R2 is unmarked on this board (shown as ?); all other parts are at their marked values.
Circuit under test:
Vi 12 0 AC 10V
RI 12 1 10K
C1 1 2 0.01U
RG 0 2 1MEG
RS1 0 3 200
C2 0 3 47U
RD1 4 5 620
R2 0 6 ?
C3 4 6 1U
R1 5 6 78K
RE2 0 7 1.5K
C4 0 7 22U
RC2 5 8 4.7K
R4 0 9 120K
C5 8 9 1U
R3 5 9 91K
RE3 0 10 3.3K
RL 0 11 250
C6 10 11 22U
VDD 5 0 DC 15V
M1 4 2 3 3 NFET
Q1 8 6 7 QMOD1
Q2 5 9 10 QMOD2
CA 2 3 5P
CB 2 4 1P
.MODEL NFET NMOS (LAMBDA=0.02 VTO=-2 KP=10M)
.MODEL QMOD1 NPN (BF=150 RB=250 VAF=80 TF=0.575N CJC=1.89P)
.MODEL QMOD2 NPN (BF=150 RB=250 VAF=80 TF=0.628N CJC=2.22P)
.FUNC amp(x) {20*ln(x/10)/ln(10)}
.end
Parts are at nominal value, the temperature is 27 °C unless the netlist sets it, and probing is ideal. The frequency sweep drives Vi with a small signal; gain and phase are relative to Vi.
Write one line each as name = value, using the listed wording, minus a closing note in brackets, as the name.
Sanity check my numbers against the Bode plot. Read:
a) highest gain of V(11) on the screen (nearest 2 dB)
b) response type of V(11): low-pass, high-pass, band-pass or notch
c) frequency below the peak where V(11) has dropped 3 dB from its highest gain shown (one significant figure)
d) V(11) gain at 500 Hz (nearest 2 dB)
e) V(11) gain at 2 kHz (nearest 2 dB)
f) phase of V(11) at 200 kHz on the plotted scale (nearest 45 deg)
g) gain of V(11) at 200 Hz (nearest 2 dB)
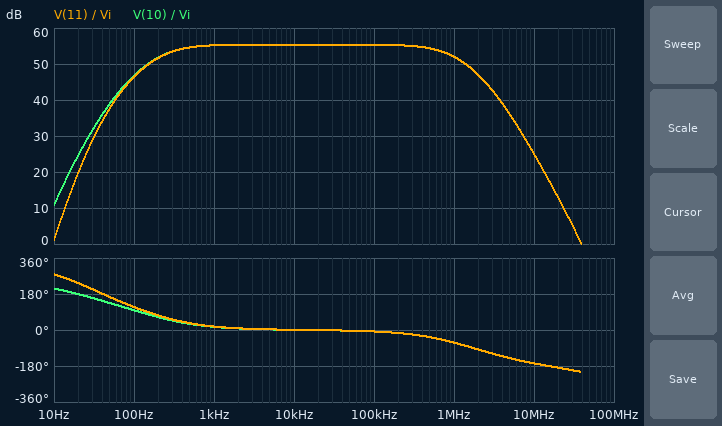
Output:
highest gain of V(11) on the screen = 56 dB
response type of V(11): low-pass, high-pass, band-pass or notch = band-pass
frequency below the peak where V(11) has dropped 3 dB from its highest gain shown = 200 Hz
V(11) gain at 500 Hz = 54 dB
V(11) gain at 2 kHz = 56 dB
phase of V(11) at 200 kHz on the plotted scale = 0 deg
gain of V(11) at 200 Hz = 52 dB
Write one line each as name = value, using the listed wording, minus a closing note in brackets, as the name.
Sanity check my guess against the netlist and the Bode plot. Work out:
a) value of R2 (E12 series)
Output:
value of R2 = 12 kΩ
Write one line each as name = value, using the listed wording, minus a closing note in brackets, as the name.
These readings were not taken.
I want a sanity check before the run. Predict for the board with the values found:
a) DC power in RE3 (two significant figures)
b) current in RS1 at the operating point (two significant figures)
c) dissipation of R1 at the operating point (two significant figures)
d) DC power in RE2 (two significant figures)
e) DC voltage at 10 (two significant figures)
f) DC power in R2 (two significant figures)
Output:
DC power in RE3 = 15 mW
current in RS1 at the operating point = 5.3 mA
dissipation of R1 at the operating point = 2.2 mW
DC power in RE2 = 940 µW
DC voltage at 10 = 7.1 V
DC power in R2 = 320 µW
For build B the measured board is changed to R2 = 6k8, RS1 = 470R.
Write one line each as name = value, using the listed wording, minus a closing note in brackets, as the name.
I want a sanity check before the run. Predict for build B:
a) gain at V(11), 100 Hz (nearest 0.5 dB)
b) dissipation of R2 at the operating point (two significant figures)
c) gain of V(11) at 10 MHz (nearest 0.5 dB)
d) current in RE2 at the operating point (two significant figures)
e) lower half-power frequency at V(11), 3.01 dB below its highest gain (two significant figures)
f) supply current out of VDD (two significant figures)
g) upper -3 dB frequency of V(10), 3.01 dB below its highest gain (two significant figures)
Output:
gain at V(11), 100 Hz = 41.5 dB
dissipation of R2 at the operating point = 210 µW
gain of V(11) at 10 MHz = 20.5 dB
current in RE2 at the operating point = 300 µA
lower half-power frequency at V(11), 3.01 dB below its highest gain = 120 Hz
supply current out of VDD = 5.5 mA
upper -3 dB frequency of V(10), 3.01 dB below its highest gain = 1.3 MHz
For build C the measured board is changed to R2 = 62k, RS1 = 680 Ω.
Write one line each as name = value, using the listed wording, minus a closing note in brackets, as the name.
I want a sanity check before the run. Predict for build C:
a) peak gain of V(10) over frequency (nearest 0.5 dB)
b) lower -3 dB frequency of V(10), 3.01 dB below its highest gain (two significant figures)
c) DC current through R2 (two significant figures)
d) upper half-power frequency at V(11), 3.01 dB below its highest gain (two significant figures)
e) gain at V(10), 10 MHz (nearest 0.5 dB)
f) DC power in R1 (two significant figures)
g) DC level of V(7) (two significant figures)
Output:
peak gain of V(10) over frequency = 8.0 dB
lower -3 dB frequency of V(10), 3.01 dB below its highest gain = 200 Hz
DC current through R2 = 72 µA
upper half-power frequency at V(11), 3.01 dB below its highest gain = 2.2 MHz
gain at V(10), 10 MHz = -5.5 dB
DC power in R1 = 1.4 mW
DC level of V(7) = 3.7 V
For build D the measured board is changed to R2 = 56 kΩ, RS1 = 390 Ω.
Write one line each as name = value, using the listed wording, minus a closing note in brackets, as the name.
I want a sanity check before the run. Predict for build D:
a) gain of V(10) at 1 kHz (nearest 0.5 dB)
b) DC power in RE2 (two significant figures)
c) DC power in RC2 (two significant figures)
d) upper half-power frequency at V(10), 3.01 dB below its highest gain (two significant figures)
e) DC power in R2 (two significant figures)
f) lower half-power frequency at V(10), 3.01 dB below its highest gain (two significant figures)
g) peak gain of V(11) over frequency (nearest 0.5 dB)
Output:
gain of V(10) at 1 kHz = 11.0 dB
DC power in RE2 = 9.0 mW
DC power in RC2 = 27 mW
upper half-power frequency at V(10), 3.01 dB below its highest gain = 2.1 MHz
DC power in R2 = 360 µW
lower half-power frequency at V(10), 3.01 dB below its highest gain = 200 Hz
peak gain of V(11) over frequency = 11.5 dB
